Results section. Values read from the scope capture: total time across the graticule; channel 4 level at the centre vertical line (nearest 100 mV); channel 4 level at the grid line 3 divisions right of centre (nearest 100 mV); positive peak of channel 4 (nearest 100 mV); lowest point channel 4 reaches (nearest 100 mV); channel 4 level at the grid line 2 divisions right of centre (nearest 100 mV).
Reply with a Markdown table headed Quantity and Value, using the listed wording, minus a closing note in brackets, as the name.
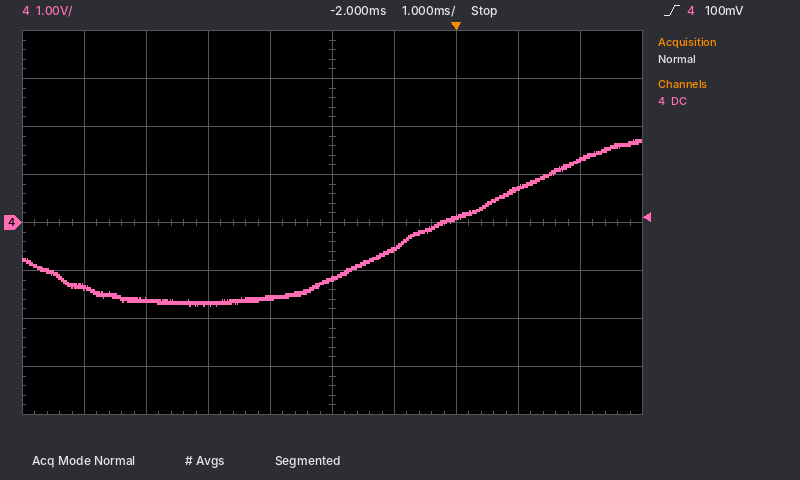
| Quantity | Value |
|---|---|
| total time across the graticule | 10 ms |
| channel 4 level at the centre vertical line | -1.2 V |
| channel 4 level at the grid line 3 divisions right of centre | 700 mV |
| positive peak of channel 4 | 1.7 V |
| lowest point channel 4 reaches | -1.7 V |
| channel 4 level at the grid line 2 divisions right of centre | 100 mV |
